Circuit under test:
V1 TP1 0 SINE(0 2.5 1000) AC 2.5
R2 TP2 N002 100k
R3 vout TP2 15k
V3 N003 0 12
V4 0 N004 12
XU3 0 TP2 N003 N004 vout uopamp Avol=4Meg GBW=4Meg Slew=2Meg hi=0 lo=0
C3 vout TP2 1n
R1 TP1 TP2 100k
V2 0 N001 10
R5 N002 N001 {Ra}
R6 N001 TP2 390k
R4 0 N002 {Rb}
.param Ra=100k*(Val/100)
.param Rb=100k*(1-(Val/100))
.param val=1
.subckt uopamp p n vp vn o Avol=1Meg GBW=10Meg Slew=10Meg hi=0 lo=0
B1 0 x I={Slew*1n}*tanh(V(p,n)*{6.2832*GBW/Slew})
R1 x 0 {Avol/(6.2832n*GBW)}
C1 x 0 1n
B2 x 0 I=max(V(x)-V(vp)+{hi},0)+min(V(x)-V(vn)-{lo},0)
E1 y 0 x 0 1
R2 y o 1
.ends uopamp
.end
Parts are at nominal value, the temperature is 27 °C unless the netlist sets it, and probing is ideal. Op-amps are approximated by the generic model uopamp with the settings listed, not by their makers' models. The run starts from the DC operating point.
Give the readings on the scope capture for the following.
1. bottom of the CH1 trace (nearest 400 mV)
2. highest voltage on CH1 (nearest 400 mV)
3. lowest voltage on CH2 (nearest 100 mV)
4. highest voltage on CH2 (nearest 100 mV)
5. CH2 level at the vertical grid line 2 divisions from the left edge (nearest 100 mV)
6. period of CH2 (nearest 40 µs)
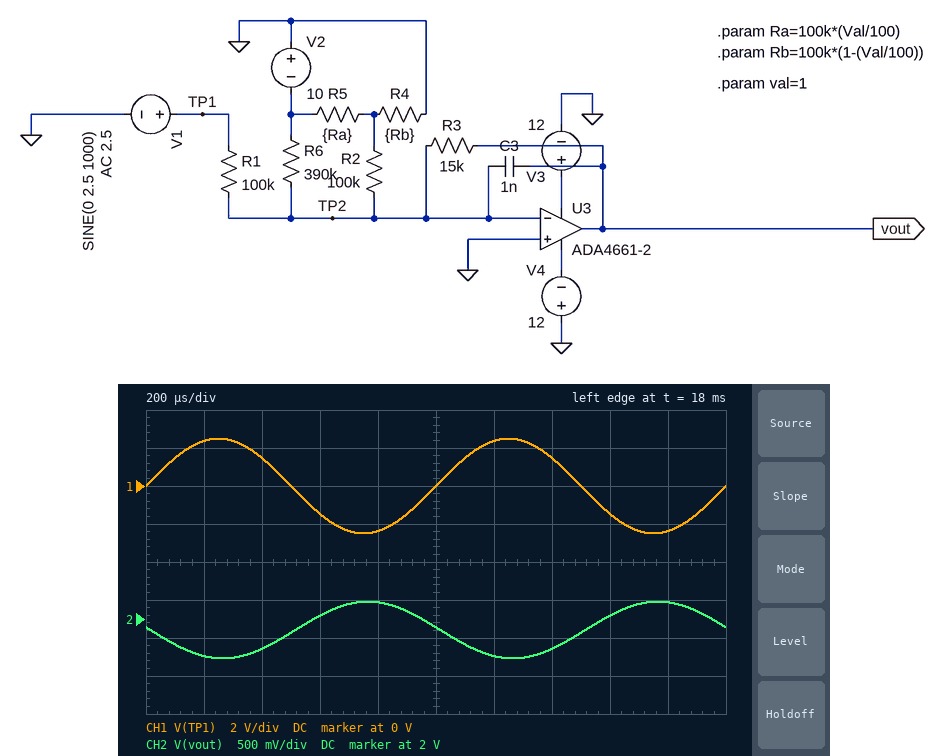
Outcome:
-2.4 V
2.4 V
1.5 V
2.2 V
1.6 V
1.00 ms
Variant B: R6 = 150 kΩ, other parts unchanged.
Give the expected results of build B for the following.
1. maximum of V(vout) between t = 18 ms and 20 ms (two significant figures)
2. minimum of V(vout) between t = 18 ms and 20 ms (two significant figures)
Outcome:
2.8 V
2.1 V
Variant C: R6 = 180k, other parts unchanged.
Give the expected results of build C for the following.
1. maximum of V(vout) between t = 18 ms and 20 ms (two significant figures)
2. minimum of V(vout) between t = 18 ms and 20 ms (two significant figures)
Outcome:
2.7 V
1.9 V
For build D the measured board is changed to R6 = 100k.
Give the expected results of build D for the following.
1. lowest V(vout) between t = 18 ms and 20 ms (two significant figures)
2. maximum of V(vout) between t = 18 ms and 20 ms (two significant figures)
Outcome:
2.6 V
3.3 V
